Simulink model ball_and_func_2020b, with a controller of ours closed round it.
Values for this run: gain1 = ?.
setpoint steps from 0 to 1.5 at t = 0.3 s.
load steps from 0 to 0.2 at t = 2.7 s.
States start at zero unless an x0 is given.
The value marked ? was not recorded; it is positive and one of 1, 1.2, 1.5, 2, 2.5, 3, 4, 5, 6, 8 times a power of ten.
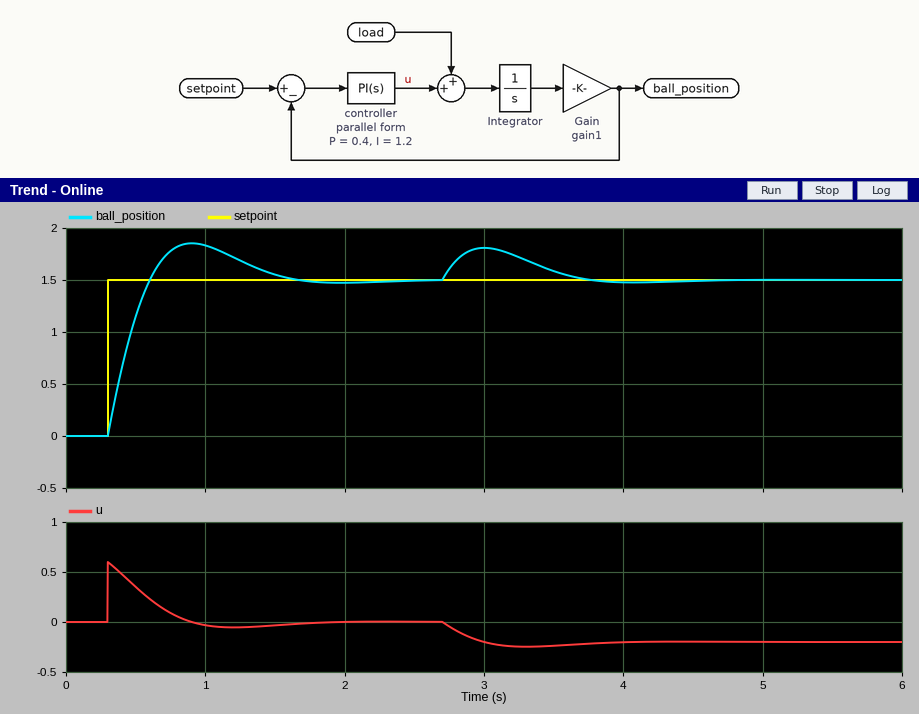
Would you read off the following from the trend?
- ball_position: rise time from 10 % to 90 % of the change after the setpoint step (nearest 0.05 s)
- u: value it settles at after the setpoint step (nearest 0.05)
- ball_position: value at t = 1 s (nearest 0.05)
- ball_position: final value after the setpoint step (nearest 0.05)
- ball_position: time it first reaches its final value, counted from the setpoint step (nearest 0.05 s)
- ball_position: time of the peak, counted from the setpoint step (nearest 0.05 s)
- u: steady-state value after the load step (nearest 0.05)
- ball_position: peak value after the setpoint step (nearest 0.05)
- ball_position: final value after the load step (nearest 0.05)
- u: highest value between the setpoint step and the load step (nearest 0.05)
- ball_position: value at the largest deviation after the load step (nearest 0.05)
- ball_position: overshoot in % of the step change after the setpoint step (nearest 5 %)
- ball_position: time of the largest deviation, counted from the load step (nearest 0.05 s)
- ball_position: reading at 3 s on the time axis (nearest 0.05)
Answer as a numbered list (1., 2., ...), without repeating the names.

1. 0.25 s
2. 0.00
3. 1.85
4. 1.50
5. 0.30 s
6. 0.60 s
7. -0.20
8. 1.85
9. 1.50
10. 0.60
11. 1.80
12. 25 %
13. 0.30 s
14. 1.80
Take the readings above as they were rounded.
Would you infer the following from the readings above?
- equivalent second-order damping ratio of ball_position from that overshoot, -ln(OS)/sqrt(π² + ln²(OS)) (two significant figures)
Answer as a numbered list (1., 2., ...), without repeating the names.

1. 0.40
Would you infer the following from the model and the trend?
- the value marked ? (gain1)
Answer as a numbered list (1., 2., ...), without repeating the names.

1. 12
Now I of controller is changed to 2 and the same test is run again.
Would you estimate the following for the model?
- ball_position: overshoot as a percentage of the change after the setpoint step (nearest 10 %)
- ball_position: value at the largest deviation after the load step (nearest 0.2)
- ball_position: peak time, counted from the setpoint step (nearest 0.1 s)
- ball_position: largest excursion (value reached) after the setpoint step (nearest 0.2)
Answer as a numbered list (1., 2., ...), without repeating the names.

1. 30 %
2. 1.8
3. 0.5 s
4. 2.0
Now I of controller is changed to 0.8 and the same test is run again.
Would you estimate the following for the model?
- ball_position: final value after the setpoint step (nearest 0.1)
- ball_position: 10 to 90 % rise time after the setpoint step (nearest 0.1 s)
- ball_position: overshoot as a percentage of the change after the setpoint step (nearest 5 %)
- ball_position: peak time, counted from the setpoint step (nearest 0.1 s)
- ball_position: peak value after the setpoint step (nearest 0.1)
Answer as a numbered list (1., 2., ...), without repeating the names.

1. 1.5
2. 0.3 s
3. 20 %
4. 0.7 s
5. 1.8
